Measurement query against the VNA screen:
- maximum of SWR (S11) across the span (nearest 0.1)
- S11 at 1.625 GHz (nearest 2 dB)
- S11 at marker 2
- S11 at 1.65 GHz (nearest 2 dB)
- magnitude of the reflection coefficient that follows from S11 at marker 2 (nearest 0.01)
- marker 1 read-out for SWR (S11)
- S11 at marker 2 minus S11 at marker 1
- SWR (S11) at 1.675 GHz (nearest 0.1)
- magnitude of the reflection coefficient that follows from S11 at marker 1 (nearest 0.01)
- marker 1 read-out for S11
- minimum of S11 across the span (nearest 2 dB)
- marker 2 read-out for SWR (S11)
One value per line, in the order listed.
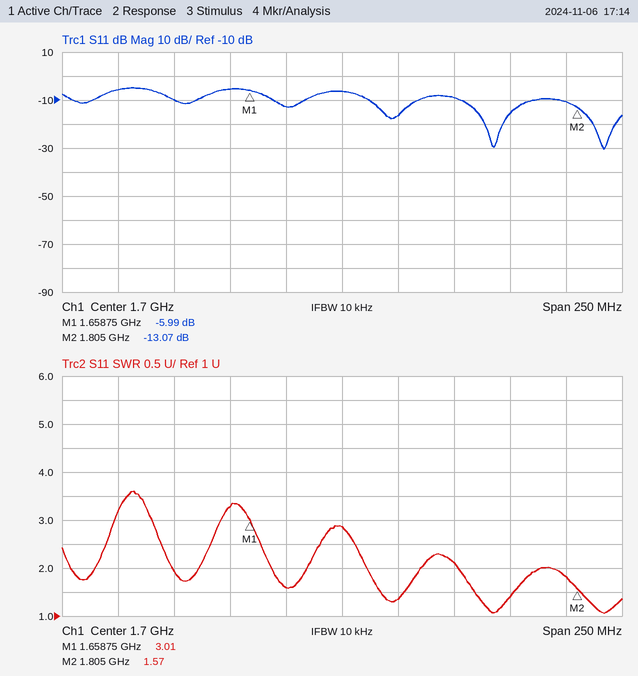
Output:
3.6
-10 dB
-13.07 dB
-6 dB
0.22
3.01
-7.08 dB
1.6
0.50
-5.99 dB
-30 dB
1.57
